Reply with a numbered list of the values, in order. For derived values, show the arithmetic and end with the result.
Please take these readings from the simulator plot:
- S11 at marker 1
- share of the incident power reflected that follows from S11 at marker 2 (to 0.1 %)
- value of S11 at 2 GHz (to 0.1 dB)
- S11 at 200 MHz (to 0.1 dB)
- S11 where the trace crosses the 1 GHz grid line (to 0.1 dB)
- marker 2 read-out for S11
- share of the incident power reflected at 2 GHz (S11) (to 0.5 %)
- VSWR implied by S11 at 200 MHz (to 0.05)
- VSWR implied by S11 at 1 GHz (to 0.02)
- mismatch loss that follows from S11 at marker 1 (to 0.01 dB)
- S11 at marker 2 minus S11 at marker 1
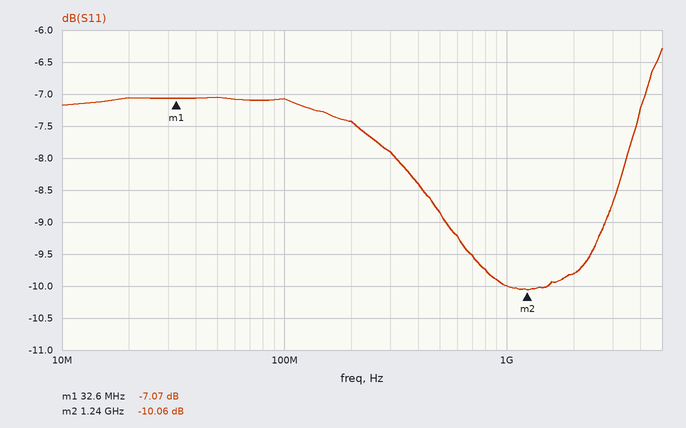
1. -7.07 dB
2. 10^(-10.06/10) ≈ 9.9 %
3. -9.8 dB
4. -7.4 dB
5. -10.0 dB
6. -10.06 dB
7. 10^(-9.8/10) ≈ 10.5 %
8. |Γ| = 10^(-7.4/20) = 0.4266; VSWR = (1 + 0.4266)/(1 − 0.4266) ≈ 2.49, so 2.50 to the nearest 0.05
9. |Γ| = 10^(-10/20) = 0.3162; VSWR = (1 + 0.3162)/(1 − 0.3162) ≈ 1.92
10. −10 log10(1 − 10^(-7.07/10)) ≈ 0.95 dB
11. -10.06 − (-7.07) = -2.99 dB
